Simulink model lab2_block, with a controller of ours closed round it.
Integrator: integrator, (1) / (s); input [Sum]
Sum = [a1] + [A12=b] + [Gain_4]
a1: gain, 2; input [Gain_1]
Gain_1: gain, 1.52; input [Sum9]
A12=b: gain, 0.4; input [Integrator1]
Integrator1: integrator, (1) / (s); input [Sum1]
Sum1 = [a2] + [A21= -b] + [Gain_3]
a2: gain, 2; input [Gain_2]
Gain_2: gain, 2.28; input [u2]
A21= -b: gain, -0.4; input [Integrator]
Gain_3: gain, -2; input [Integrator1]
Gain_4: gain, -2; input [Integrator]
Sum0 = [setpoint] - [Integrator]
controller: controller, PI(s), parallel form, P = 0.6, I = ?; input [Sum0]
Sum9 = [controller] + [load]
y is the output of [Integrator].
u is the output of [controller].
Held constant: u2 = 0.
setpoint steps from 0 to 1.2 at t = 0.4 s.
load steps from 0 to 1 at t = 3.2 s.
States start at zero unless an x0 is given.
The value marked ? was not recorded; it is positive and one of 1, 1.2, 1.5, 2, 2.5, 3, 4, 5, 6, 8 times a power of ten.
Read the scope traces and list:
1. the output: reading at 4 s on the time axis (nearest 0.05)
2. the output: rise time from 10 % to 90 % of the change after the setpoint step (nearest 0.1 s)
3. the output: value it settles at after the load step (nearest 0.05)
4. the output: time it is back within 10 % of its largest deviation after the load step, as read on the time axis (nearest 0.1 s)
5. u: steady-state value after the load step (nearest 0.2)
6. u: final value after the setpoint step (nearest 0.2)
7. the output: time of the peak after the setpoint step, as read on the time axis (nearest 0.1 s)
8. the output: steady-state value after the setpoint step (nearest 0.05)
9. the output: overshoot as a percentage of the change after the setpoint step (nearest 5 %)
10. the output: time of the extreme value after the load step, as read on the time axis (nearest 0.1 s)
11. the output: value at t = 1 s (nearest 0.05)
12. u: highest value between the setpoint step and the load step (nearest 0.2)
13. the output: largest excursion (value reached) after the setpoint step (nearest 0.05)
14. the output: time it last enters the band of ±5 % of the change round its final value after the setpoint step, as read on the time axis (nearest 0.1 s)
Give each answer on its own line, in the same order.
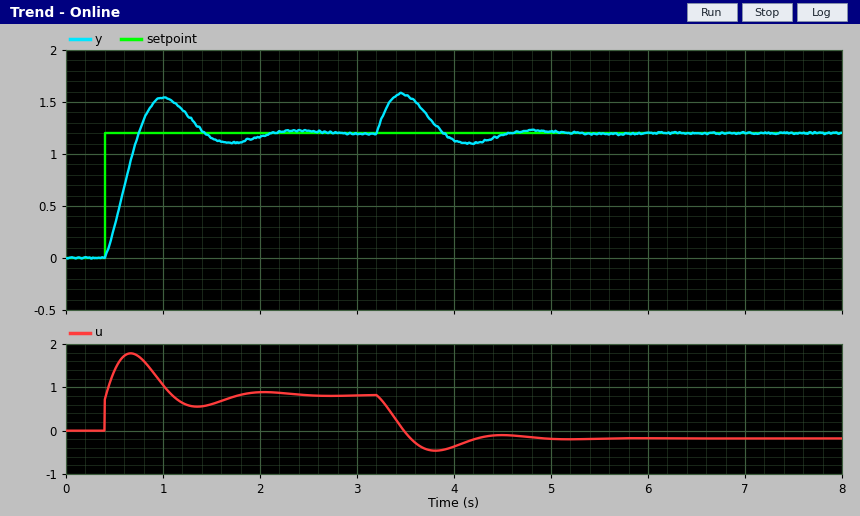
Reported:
1.15
0.3 s
1.20
4.4 s
-0.2
0.8
1.0 s
1.20
30 %
3.5 s
1.55
1.8
1.55
1.9 s
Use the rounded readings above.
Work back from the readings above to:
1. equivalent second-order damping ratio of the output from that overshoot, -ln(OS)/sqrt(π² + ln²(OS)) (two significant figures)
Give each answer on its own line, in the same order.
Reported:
0.36
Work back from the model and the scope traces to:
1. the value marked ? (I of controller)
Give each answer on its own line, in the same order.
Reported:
8
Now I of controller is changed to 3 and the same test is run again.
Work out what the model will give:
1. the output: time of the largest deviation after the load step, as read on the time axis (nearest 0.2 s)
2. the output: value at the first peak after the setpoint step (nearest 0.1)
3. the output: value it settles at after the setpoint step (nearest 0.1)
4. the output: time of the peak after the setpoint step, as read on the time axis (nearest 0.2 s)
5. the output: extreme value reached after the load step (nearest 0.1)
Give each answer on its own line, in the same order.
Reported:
3.6 s
1.3
1.2
1.4 s
1.7
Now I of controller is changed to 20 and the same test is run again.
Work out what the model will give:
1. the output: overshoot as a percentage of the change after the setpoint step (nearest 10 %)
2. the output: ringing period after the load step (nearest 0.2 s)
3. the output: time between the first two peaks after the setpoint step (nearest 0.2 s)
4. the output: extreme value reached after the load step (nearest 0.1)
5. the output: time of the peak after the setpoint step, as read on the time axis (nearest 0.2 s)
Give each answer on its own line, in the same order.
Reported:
50 %
0.8 s
0.8 s
1.5
0.8 s
